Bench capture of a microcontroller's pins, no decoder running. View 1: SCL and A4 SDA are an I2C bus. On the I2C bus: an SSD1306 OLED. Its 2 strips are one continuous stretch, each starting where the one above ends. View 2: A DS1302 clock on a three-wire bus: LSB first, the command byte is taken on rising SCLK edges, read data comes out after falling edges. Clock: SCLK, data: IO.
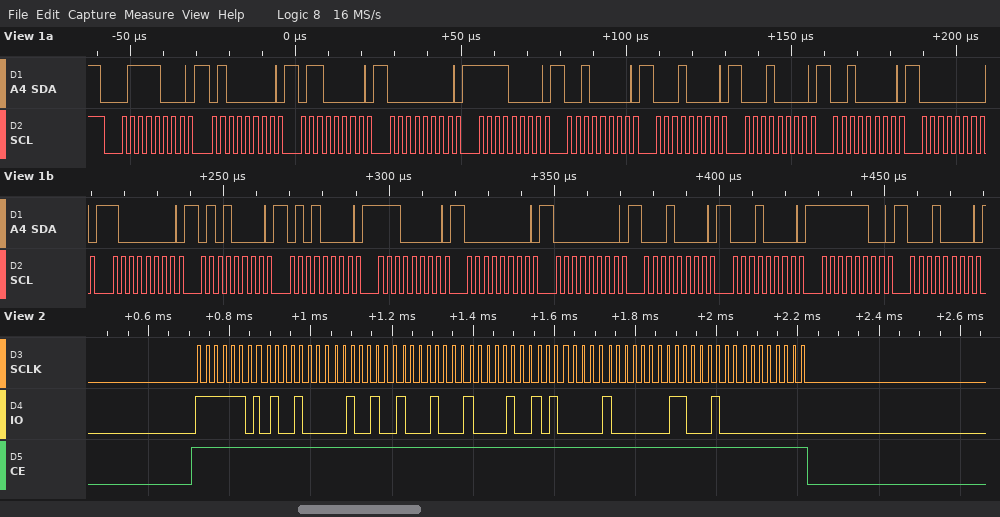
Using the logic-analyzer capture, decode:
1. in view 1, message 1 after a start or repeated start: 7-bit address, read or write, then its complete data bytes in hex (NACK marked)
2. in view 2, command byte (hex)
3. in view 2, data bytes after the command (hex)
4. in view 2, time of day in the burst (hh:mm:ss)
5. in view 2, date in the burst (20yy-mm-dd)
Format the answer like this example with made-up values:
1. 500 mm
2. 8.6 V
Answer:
1. 0x3C write: 40 60 00 F0 20 10 10 20 00 80 50 50 E0 00 00 10 10 FC 10
2. 0xBF
3. 12 24 11 21 05 01 23 00
4. 11:24:12
5. 2023-05-21
